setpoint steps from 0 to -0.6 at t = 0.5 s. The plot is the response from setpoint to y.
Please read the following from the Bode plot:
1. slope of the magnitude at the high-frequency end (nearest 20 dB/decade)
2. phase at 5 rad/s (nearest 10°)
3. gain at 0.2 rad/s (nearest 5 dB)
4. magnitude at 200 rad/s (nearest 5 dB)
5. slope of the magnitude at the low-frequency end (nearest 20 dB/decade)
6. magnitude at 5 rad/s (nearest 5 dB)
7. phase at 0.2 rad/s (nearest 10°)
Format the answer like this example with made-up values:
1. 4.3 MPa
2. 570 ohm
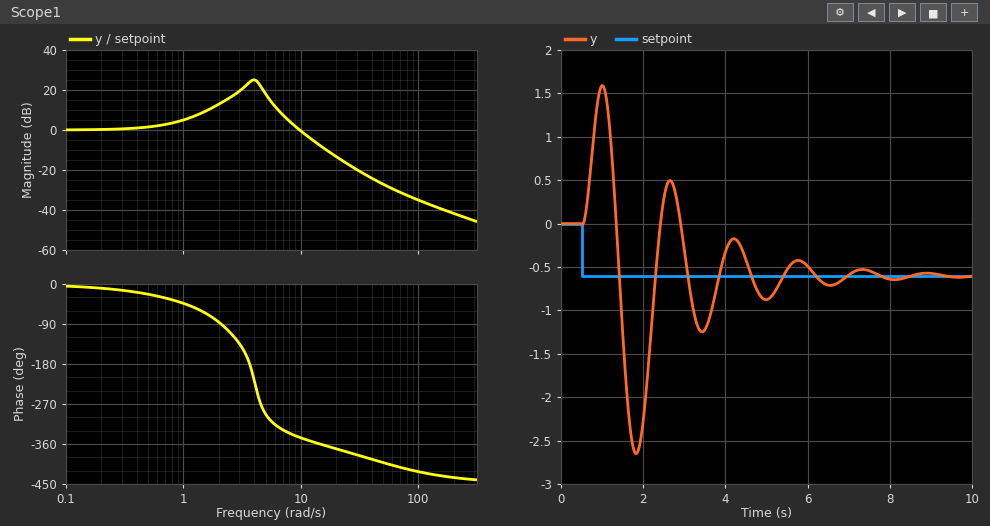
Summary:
1. -20 dB/decade
2. -290°
3. 0 dB
4. -40 dB
5. 0 dB/decade
6. 20 dB
7. -10°
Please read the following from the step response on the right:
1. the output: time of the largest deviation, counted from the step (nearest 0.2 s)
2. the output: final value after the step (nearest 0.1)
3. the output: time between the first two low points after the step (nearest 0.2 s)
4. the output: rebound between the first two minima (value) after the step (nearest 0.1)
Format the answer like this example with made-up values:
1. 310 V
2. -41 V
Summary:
1. 1.4 s
2. -0.6
3. 1.6 s
4. 0.5
